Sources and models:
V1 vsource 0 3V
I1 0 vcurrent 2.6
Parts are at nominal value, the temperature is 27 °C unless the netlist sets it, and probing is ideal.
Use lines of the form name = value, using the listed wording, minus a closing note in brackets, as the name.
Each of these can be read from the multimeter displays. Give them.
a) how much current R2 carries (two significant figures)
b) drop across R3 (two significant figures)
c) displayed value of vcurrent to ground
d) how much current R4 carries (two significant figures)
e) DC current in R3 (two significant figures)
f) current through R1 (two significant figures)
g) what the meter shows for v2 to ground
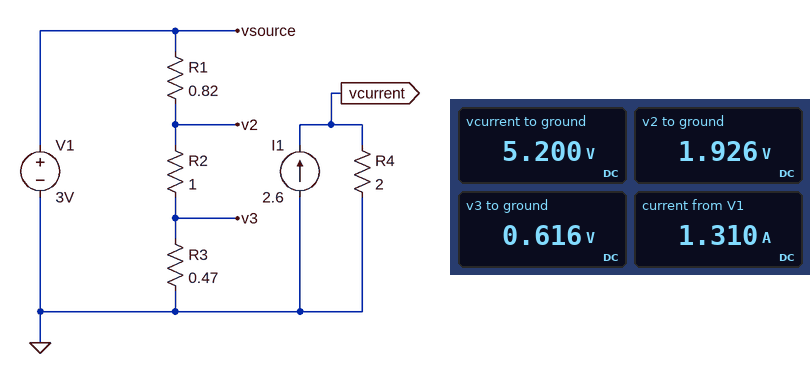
how much current R2 carries = 1.3 A
drop across R3 = 620 mV
displayed value of vcurrent to ground = 5.200 V
how much current R4 carries = 2.6 A
DC current in R3 = 1.3 A
current through R1 = 1.3 A
what the meter shows for v2 to ground = 1.926 V
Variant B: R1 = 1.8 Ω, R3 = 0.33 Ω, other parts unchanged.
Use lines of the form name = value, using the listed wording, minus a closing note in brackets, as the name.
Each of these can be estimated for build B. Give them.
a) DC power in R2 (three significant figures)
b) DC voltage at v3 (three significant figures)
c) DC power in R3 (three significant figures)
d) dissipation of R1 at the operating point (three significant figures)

DC power in R2 = 919 mW
DC voltage at v3 = 316 mV
DC power in R3 = 303 mW
dissipation of R1 at the operating point = 1.65 W
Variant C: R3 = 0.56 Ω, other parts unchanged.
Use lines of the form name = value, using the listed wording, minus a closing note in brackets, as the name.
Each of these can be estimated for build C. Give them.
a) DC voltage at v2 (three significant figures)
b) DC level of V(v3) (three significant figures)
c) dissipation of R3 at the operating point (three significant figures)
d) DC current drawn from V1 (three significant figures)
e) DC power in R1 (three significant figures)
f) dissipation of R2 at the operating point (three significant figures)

DC voltage at v2 = 1.97 V
DC level of V(v3) = 706 mV
dissipation of R3 at the operating point = 890 mW
DC current drawn from V1 = 1.26 A
DC power in R1 = 1.30 W
dissipation of R2 at the operating point = 1.59 W
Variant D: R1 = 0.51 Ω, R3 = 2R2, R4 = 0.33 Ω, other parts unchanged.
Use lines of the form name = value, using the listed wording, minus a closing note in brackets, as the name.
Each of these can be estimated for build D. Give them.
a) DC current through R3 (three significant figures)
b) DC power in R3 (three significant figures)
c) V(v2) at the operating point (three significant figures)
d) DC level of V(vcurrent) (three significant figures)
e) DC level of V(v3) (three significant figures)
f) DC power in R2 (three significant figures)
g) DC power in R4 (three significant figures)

DC current through R3 = 809 mA
DC power in R3 = 1.44 W
V(v2) at the operating point = 2.59 V
DC level of V(vcurrent) = 858 mV
DC level of V(v3) = 1.78 V
DC power in R2 = 654 mW
DC power in R4 = 2.23 W
